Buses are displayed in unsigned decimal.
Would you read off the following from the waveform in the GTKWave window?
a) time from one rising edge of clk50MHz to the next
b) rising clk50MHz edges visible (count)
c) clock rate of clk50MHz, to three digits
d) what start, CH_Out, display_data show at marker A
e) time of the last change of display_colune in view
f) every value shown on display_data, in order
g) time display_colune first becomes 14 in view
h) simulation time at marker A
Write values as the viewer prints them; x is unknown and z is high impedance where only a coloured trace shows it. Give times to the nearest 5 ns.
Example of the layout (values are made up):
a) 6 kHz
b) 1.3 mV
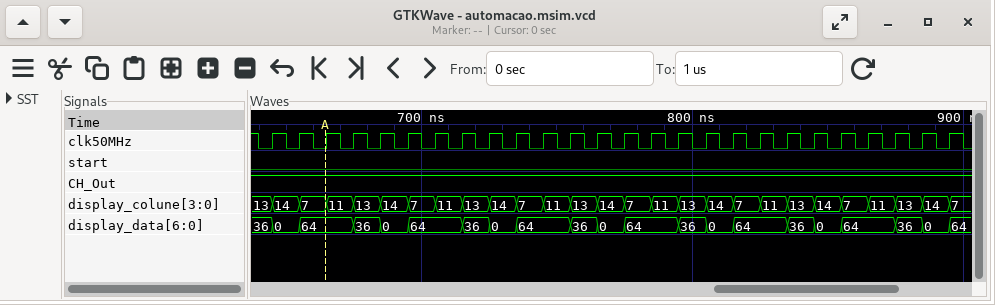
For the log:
a) 10 ns
b) 26
c) 100 MHz
d) start=0, CH_Out=1, display_data=64
e) 895 ns
f) 36, 0, 64, 36, 0, 64, 36, 0, 64, 36, 0, 64, 36, 0, 64, 36, 0, 64, 36, 0, 64
g) 645 ns
h) 665 ns
